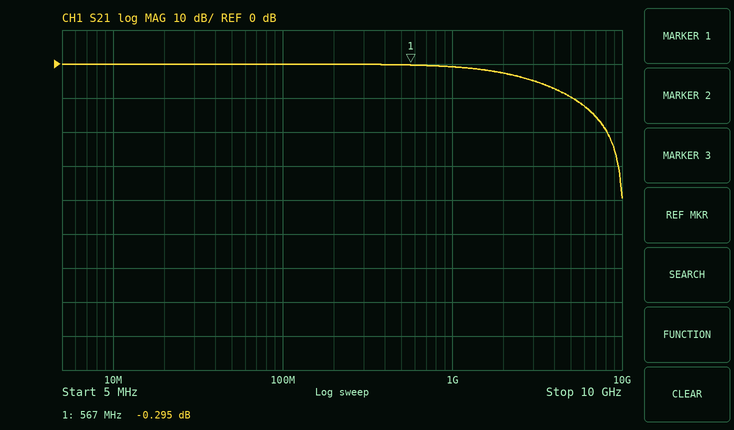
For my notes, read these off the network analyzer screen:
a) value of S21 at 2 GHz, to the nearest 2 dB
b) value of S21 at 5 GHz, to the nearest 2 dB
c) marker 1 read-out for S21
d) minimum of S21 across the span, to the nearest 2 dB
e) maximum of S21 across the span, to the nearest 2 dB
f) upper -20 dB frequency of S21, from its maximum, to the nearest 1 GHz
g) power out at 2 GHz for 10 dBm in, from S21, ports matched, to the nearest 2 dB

-2 dB
-10 dB
-0.295 dB
-40 dB
0 dB
8 GHz
8 dBm
